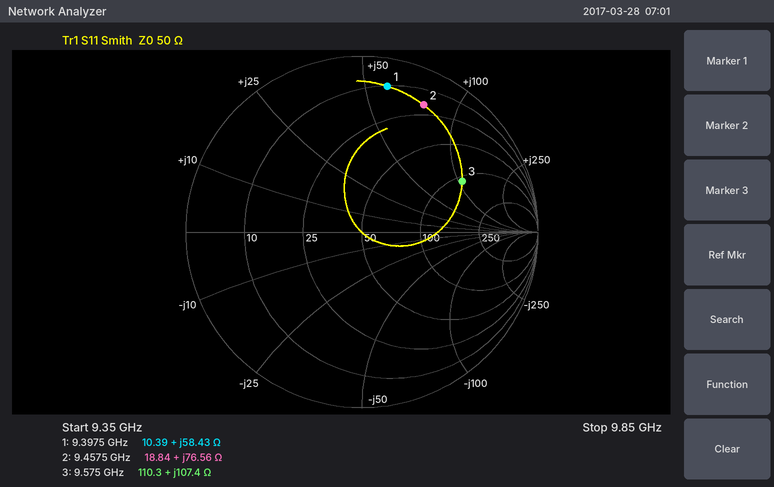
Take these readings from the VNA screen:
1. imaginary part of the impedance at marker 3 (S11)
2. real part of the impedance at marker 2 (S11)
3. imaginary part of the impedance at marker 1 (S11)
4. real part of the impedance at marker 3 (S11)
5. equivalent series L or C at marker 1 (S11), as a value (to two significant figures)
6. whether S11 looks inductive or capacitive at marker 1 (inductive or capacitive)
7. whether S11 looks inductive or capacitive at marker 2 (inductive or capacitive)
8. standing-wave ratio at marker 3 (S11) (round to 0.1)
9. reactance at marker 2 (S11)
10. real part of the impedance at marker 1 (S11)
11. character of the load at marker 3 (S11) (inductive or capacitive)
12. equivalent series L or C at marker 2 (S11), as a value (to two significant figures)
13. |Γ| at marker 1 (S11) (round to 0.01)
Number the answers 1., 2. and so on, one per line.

1. +107.4 Ω
2. 18.84 Ω
3. +58.43 Ω
4. 110.3 Ω
5. 990 pH
6. inductive
7. inductive
8. 4.5
9. +76.56 Ω
10. 10.39 Ω
11. inductive
12. 1.3 nH
13. 0.84
